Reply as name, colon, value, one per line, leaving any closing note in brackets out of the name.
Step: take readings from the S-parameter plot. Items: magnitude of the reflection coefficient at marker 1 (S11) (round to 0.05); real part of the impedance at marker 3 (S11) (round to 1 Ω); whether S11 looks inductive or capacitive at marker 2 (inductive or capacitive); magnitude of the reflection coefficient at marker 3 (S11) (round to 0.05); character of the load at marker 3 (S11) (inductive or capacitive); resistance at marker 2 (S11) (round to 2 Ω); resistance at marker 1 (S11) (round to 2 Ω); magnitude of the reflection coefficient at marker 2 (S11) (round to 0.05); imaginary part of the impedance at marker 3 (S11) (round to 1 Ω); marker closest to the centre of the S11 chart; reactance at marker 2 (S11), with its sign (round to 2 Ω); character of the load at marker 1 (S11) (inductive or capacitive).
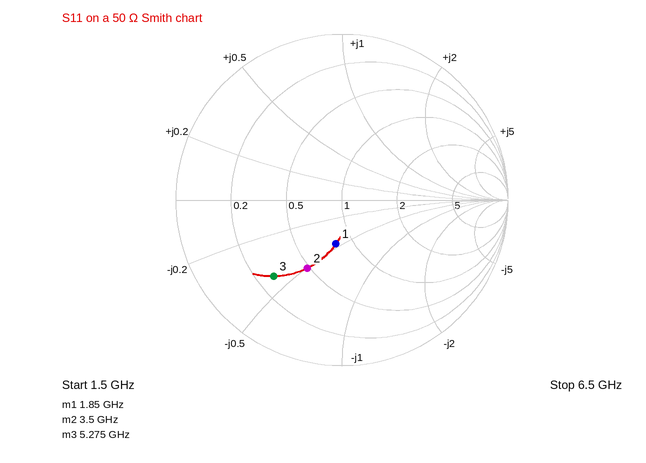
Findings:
magnitude of the reflection coefficient at marker 1 (S11): 0.25
real part of the impedance at marker 3 (S11): 14 Ω
whether S11 looks inductive or capacitive at marker 2: capacitive
magnitude of the reflection coefficient at marker 3 (S11): 0.60
character of the load at marker 3 (S11): capacitive
resistance at marker 2 (S11): 24 Ω
resistance at marker 1 (S11): 40 Ω
magnitude of the reflection coefficient at marker 2 (S11): 0.45
imaginary part of the impedance at marker 3 (S11): -21 Ω
marker closest to the centre of the S11 chart: marker 1
reactance at marker 2 (S11), with its sign: -26 Ω
character of the load at marker 1 (S11): capacitive
